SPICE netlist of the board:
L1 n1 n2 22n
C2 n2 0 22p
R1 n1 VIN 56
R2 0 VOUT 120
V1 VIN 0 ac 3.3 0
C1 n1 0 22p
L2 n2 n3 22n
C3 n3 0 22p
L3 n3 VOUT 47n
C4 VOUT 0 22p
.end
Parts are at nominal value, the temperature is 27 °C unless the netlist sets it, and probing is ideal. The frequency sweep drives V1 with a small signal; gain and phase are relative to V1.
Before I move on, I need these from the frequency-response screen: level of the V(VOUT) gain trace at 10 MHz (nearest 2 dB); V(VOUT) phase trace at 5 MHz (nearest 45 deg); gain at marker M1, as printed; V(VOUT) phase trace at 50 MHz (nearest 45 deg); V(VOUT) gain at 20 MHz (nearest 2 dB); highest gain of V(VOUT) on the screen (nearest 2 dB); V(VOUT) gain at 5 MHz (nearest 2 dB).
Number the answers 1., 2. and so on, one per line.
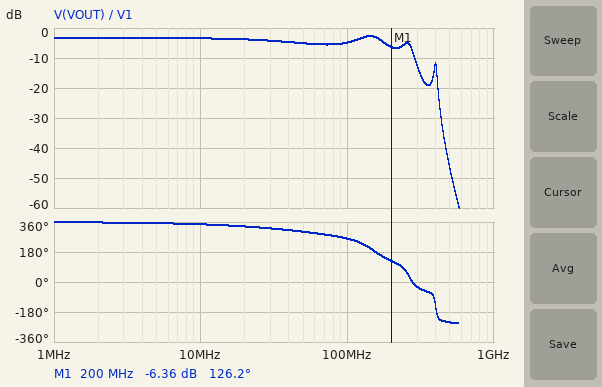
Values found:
1. -4 dB
2. 360 deg
3. -6.36 dB
4. 315 deg
5. -4 dB
6. -2 dB
7. -4 dB
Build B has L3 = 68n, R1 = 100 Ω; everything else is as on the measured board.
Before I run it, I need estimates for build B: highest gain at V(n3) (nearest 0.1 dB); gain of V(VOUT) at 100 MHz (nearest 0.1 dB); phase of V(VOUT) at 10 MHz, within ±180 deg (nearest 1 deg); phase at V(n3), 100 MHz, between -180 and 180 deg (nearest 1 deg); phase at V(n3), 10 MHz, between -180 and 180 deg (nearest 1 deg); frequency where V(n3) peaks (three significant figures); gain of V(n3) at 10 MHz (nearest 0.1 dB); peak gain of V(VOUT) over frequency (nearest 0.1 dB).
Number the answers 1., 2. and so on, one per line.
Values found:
1. 1.8 dB
2. -7.8 dB
3. -19 deg
4. -70 deg
5. -17 deg
6. 399 MHz
7. -5.6 dB
8. -5.3 dB
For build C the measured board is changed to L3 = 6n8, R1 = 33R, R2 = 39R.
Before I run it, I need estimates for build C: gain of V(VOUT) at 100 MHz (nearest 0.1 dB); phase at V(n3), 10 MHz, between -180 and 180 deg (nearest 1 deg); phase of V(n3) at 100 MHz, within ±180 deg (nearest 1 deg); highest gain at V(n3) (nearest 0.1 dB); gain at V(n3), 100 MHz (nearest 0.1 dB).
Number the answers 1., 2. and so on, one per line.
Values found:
1. -5.6 dB
2. -8 deg
3. -72 deg
4. -5.3 dB
5. -6.1 dB
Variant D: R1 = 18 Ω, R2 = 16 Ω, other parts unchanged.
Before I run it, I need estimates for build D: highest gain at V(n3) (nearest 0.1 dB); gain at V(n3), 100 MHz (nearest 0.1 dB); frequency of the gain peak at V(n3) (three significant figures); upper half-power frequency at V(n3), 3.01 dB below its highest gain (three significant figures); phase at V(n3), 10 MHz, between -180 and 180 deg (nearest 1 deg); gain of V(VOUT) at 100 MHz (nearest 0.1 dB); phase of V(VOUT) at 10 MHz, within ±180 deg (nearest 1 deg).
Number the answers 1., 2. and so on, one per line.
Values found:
1. 7.4 dB
2. -3.6 dB
3. 387 MHz
4. 398 MHz
5. -2 deg
6. -9.3 dB
7. -12 deg
